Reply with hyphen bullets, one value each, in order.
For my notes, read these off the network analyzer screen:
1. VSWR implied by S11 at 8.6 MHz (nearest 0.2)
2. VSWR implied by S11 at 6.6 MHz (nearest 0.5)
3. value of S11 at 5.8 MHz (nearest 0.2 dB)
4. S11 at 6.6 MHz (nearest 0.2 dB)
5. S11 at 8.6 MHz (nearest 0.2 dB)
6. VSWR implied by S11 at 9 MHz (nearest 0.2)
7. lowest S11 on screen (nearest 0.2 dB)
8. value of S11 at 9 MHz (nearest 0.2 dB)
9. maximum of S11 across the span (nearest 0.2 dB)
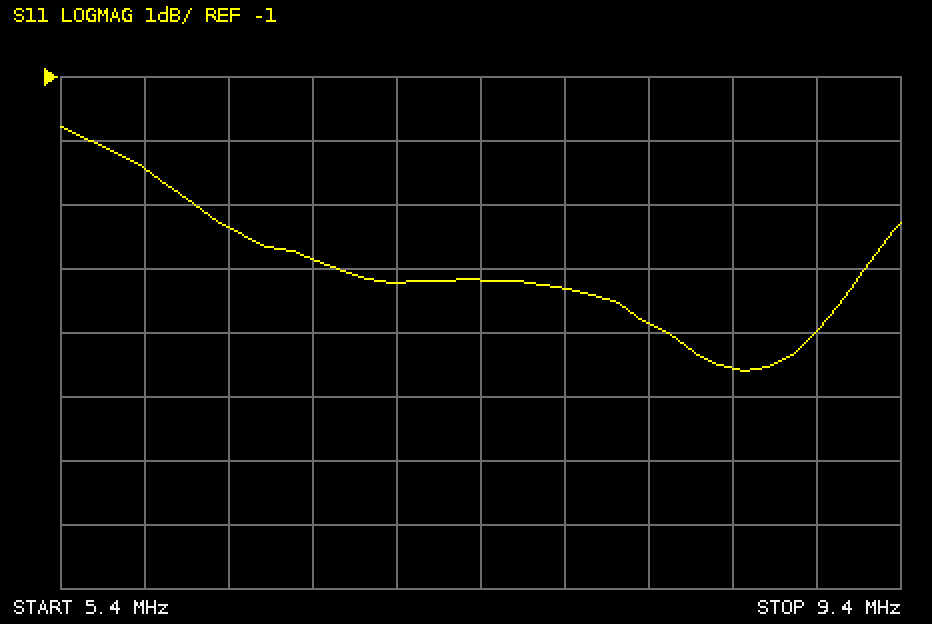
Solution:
- 3.2
- 4.5
- -2.4 dB
- -3.8 dB
- -5.6 dB
- 3.6
- -5.6 dB
- -5.0 dB
- -1.8 dB
